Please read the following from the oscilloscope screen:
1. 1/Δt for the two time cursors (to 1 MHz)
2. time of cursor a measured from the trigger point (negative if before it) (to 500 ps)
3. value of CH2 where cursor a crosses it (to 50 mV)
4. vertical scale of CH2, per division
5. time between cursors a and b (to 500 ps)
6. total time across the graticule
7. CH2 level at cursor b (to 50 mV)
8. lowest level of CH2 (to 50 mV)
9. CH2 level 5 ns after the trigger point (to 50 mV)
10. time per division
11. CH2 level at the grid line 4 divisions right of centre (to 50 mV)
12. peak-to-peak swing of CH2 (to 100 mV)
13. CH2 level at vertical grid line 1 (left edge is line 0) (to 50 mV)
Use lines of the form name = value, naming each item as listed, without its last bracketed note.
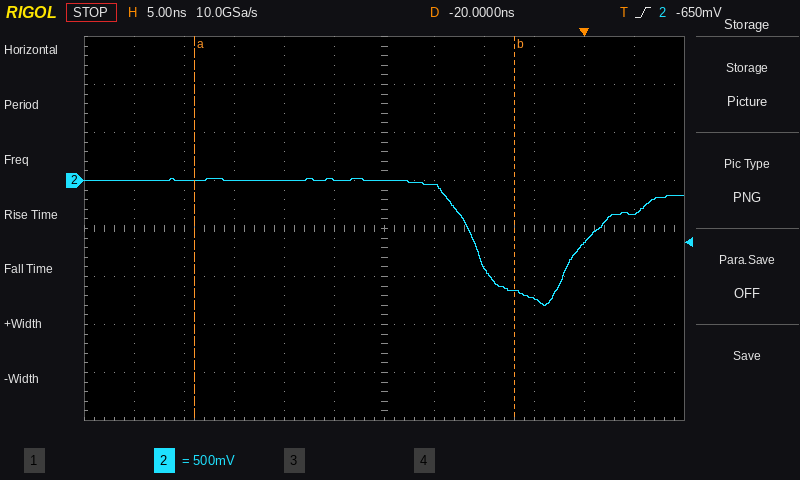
1/Δt for the two time cursors = 31 MHz
time of cursor a measured from the trigger point (negative if before it) = -39.0 ns
value of CH2 where cursor a crosses it = 0 mV
vertical scale of CH2, per division = 500 mV
time between cursors a and b = 32.0 ns
total time across the graticule = 60 ns
CH2 level at cursor b = -1.15 V
lowest level of CH2 = -1.30 V
CH2 level 5 ns after the trigger point = -350 mV
time per division = 5 ns
CH2 level at the grid line 4 divisions right of centre = -650 mV
peak-to-peak swing of CH2 = 1.30 V
CH2 level at vertical grid line 1 (left edge is line 0) = 0 mV
